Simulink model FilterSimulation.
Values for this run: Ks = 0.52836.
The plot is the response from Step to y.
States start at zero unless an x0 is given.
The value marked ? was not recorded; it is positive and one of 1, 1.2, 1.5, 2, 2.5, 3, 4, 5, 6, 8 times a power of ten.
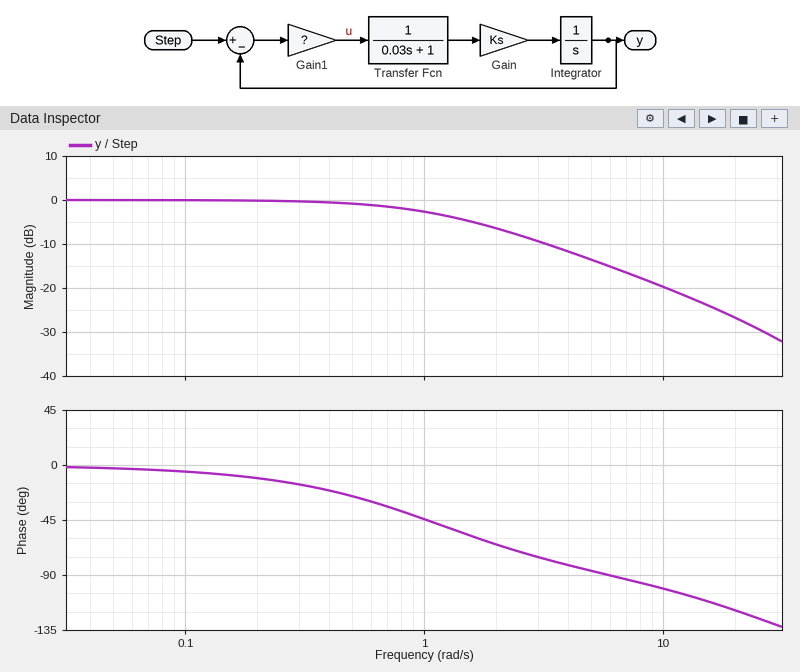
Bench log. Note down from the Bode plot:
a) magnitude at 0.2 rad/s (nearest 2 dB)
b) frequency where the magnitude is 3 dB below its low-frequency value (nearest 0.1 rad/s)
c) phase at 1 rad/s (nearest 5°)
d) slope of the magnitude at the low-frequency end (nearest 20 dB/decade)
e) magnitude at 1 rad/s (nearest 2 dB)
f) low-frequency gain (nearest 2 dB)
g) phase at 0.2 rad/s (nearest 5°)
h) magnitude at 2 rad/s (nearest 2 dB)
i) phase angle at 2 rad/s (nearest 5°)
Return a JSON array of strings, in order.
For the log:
["0 dB", "1.1 rad/s", "-45°", "0 dB/decade", "-2 dB", "0 dB", "-10°", "-6 dB", "-65°"]
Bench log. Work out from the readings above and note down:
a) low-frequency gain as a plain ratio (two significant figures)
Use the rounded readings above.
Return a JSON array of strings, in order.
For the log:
["1.0"]
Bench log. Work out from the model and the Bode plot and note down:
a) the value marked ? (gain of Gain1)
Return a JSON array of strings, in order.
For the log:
["2"]
